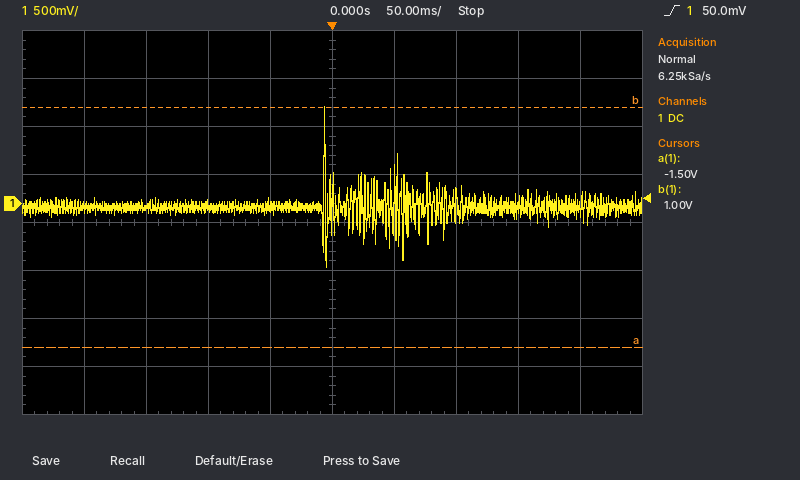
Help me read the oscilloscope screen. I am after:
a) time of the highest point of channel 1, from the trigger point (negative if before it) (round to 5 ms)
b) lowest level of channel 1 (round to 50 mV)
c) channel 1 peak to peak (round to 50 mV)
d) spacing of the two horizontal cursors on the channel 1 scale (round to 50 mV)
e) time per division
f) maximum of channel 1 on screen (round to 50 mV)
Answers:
-5 ms
-650 mV
1.65 V
2.50 V
50 ms
1.00 V
